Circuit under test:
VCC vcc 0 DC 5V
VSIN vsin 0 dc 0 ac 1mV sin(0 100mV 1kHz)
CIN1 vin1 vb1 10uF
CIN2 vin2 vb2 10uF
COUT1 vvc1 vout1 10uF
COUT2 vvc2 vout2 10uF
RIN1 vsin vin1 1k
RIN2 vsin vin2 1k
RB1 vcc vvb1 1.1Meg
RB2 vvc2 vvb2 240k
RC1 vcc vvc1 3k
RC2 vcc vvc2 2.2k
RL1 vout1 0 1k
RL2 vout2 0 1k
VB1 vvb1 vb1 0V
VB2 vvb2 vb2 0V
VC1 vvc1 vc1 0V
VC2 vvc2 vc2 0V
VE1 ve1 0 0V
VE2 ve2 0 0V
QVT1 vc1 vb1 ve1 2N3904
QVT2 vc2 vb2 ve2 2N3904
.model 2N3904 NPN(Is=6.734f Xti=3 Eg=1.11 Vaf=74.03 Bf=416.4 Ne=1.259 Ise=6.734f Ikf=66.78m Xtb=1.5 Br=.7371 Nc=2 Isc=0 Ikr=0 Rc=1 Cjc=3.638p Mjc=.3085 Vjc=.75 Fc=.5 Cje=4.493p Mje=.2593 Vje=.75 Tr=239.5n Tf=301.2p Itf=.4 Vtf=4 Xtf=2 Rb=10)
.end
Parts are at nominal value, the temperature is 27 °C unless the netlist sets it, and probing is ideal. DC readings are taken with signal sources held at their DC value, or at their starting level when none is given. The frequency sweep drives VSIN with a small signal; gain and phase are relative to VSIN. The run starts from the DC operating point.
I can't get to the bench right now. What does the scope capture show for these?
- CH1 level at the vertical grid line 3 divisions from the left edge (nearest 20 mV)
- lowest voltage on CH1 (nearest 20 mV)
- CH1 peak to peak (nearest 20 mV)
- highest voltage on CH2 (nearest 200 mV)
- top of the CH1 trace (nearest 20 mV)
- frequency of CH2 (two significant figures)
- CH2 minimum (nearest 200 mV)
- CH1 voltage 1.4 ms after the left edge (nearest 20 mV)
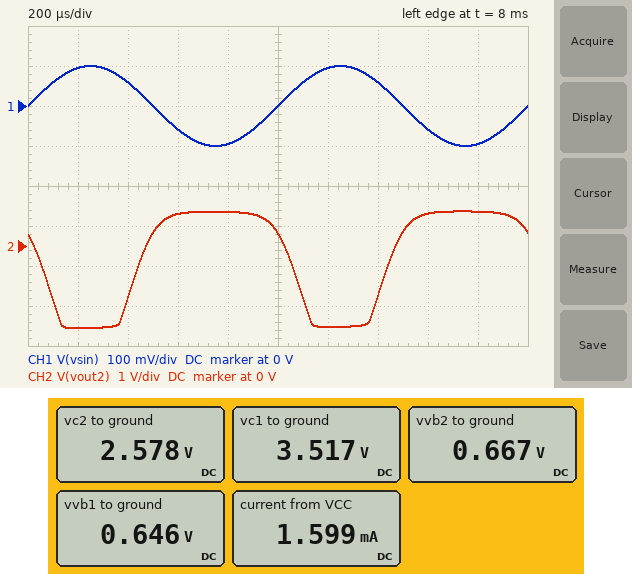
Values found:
-60 mV
-100 mV
200 mV
800 mV
100 mV
1.0 kHz
-2.0 V
60 mV
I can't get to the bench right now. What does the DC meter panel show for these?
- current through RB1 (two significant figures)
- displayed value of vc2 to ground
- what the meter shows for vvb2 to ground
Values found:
4.0 µA
2.578 V
0.667 V
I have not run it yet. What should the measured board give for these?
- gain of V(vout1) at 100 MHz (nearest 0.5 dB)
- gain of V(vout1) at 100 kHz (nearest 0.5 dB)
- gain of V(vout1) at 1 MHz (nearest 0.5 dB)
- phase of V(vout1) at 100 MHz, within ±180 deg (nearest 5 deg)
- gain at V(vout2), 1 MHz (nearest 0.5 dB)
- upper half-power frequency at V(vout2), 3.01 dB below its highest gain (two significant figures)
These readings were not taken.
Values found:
-7.0 dB
22.0 dB
21.5 dB
75 deg
25.5 dB
2.4 MHz
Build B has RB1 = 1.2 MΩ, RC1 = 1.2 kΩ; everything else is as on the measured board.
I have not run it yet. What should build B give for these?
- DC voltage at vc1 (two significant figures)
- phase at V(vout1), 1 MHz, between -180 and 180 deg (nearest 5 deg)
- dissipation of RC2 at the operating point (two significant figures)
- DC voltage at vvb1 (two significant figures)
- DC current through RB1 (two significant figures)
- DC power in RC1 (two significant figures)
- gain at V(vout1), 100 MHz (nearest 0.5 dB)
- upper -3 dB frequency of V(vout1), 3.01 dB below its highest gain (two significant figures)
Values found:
4.5 V
170 deg
2.7 mW
640 mV
3.6 µA
250 µW
-7.5 dB
5.2 MHz
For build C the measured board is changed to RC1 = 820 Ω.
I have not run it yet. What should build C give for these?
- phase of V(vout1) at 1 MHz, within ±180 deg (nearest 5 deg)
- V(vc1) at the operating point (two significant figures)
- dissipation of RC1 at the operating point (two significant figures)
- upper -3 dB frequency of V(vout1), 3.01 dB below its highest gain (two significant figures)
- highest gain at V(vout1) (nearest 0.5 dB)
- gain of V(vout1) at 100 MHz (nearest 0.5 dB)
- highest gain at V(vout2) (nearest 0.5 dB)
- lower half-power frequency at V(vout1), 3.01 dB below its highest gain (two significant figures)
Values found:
170 deg
4.6 V
210 µW
5.4 MHz
17.5 dB
-8.0 dB
26.0 dB
9.1 Hz
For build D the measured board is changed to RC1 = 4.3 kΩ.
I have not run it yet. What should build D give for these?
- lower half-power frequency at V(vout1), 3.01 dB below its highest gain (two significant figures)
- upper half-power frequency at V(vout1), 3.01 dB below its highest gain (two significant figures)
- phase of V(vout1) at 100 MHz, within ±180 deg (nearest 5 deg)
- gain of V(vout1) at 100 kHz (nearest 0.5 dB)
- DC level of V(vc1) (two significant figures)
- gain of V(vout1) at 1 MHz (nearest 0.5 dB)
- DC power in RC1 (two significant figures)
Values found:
3.9 Hz
3.4 MHz
70 deg
22.5 dB
2.9 V
22.0 dB
1.0 mW
